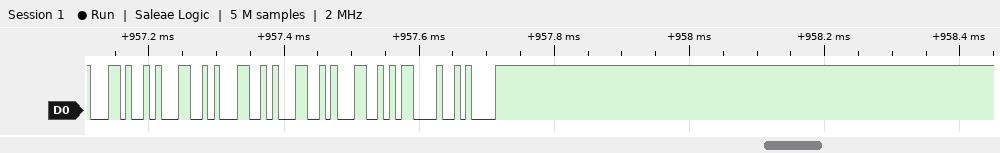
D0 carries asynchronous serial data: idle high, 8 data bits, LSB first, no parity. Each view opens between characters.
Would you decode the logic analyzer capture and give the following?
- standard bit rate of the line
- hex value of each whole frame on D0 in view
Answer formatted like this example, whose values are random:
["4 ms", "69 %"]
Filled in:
["115200 baud", "2C, 31, 31, 31, 31, 0D, 0A"]
